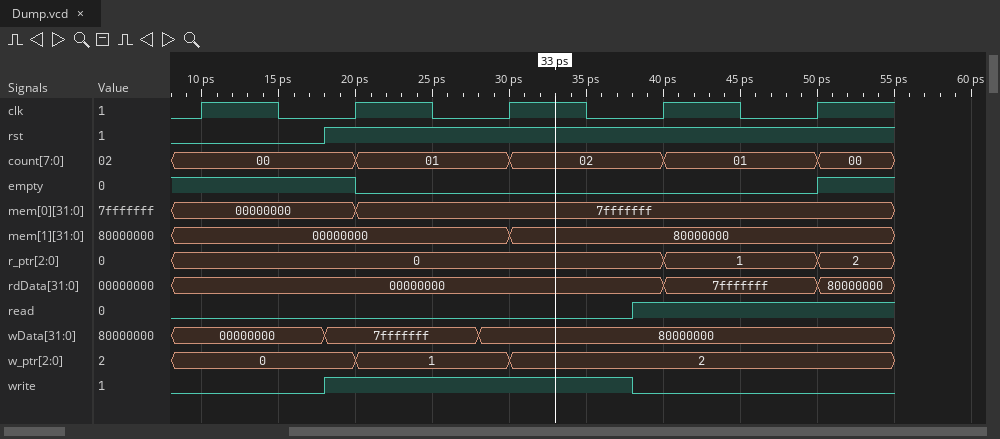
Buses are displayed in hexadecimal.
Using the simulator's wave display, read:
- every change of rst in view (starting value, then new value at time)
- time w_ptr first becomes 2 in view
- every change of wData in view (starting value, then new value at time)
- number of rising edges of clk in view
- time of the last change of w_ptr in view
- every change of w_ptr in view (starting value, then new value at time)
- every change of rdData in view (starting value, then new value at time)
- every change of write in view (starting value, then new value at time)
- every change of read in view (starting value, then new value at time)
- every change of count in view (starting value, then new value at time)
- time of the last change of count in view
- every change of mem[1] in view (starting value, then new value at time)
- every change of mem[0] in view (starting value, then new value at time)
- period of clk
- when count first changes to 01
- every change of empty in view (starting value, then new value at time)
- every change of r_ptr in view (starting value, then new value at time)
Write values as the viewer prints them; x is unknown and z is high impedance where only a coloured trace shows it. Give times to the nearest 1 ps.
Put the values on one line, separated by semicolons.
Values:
0, 1 at 18 ps; 30 ps; 00000000, 7fffffff at 18 ps, 80000000 at 28 ps; 5; 30 ps; 0, 1 at 20 ps, 2 at 30 ps; 00000000, 7fffffff at 40 ps, 80000000 at 50 ps; 0, 1 at 18 ps, 0 at 38 ps; 0, 1 at 38 ps; 00, 01 at 20 ps, 02 at 30 ps, 01 at 40 ps, 00 at 50 ps; 50 ps; 00000000, 80000000 at 30 ps; 00000000, 7fffffff at 20 ps; 10 ps; 20 ps; 1, 0 at 20 ps, 1 at 50 ps; 0, 1 at 40 ps, 2 at 50 ps
